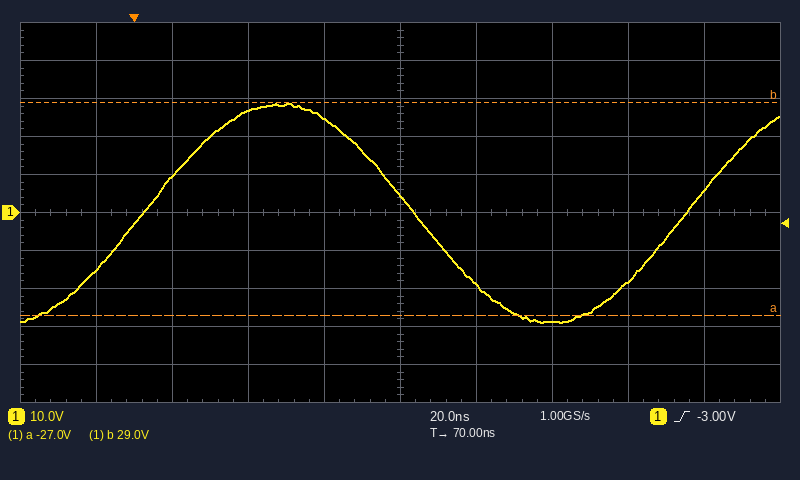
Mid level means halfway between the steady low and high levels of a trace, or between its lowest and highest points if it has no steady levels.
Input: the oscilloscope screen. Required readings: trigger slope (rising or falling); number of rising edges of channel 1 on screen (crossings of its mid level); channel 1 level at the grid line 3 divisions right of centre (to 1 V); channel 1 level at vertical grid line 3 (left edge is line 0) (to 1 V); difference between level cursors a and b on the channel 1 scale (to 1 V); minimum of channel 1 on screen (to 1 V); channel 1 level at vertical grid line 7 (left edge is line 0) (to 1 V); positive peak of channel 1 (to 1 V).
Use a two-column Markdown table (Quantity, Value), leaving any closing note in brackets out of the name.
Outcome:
| Quantity | Value |
|---|---|
| trigger slope | rising |
| number of rising edges of channel 1 on screen | 2 |
| channel 1 level at the grid line 3 divisions right of centre | -18 V |
| channel 1 level at vertical grid line 3 (left edge is line 0) | 27 V |
| difference between level cursors a and b on the channel 1 scale | 56 V |
| minimum of channel 1 on screen | -29 V |
| channel 1 level at vertical grid line 7 (left edge is line 0) | -29 V |
| positive peak of channel 1 | 29 V |
